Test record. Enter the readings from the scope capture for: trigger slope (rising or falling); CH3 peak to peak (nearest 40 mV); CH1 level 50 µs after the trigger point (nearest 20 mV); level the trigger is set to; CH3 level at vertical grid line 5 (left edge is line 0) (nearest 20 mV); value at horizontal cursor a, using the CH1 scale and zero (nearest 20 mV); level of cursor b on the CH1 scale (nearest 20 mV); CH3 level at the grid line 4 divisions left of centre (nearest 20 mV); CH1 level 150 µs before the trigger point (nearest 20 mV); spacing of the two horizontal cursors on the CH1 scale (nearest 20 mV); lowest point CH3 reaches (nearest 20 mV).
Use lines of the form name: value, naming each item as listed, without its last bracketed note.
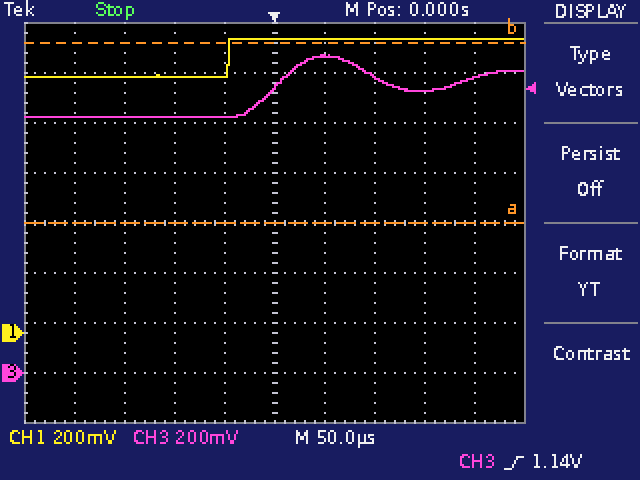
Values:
trigger slope: rising
CH3 peak to peak: 240 mV
CH1 level 50 µs after the trigger point: 1.18 V
level the trigger is set to: 1.14 V
CH3 level at vertical grid line 5 (left edge is line 0): 1.14 V
value at horizontal cursor a, using the CH1 scale and zero: 440 mV
level of cursor b on the CH1 scale: 1.16 V
CH3 level at the grid line 4 divisions left of centre: 1.02 V
CH1 level 150 µs before the trigger point: 1.02 V
spacing of the two horizontal cursors on the CH1 scale: 720 mV
lowest point CH3 reaches: 1.02 V
